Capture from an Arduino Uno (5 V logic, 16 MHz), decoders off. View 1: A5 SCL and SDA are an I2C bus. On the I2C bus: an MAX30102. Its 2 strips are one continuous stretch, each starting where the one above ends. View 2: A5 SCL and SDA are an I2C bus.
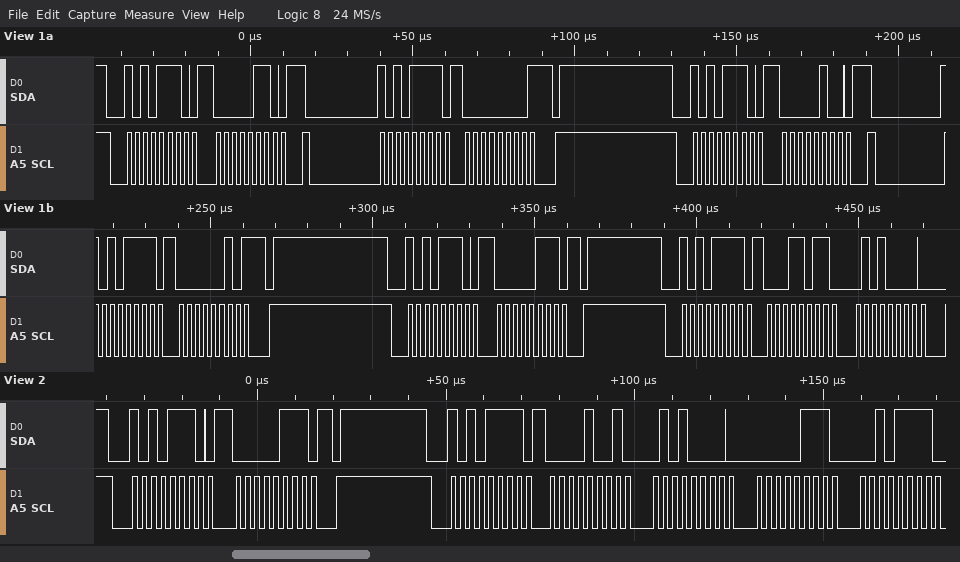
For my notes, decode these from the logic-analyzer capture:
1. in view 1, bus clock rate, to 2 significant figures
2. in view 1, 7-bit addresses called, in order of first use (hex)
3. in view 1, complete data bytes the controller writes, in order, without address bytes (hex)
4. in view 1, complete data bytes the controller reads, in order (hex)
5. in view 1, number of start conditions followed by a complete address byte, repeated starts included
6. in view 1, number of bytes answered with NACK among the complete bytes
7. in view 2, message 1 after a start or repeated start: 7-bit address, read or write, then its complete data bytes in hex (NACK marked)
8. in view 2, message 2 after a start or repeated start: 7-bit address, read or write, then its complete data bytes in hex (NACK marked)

400 kHz
0x57
06 04 07
00 02 1B 50
6
2
0x57 write: 07
0x57 read: 09 50 07 2F
